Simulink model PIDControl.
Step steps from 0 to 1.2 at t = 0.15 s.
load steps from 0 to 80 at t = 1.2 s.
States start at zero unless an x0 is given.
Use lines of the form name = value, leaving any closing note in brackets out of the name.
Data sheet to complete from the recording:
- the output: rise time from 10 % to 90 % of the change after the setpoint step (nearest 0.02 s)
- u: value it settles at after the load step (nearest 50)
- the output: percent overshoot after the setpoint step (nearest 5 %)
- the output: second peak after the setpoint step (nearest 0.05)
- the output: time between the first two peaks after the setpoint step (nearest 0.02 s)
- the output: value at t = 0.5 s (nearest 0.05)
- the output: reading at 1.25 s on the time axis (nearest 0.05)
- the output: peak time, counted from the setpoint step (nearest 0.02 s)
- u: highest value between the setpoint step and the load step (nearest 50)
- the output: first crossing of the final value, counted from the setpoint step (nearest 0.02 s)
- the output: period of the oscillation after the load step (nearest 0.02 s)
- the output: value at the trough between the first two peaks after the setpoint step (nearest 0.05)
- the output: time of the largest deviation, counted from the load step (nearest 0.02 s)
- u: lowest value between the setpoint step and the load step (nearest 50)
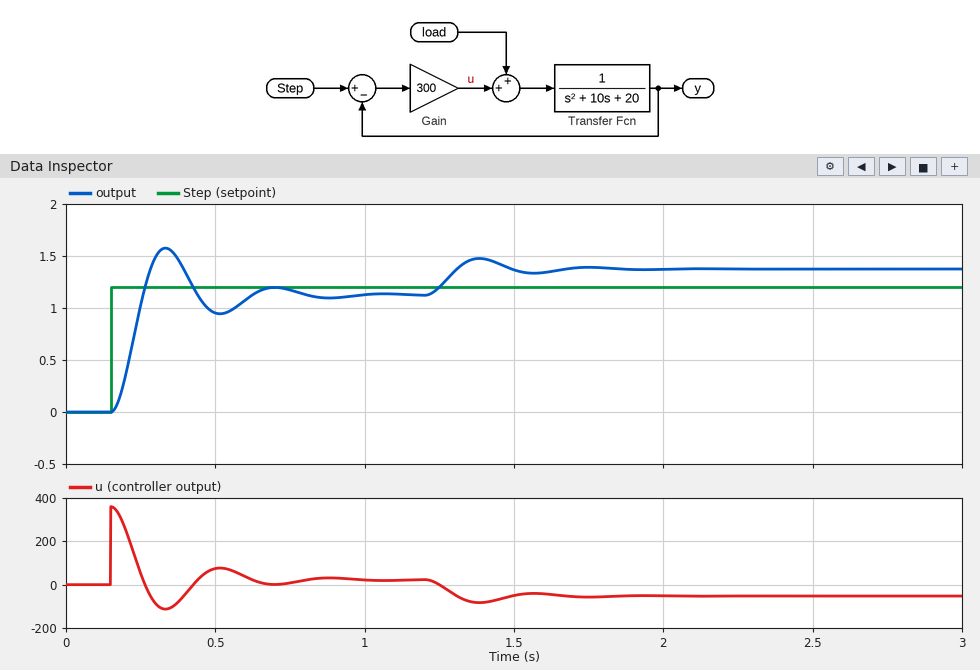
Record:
the output: rise time from 10 % to 90 % of the change after the setpoint step = 0.08 s
u: value it settles at after the load step = -50
the output: percent overshoot after the setpoint step = 40 %
the output: second peak after the setpoint step = 1.20
the output: time between the first two peaks after the setpoint step = 0.36 s
the output: value at t = 0.5 s = 0.95
the output: reading at 1.25 s on the time axis = 1.20
the output: peak time, counted from the setpoint step = 0.18 s
u: highest value between the setpoint step and the load step = 350
the output: first crossing of the final value, counted from the setpoint step = 0.10 s
the output: period of the oscillation after the load step = 0.36 s
the output: value at the trough between the first two peaks after the setpoint step = 0.95
the output: time of the largest deviation, counted from the load step = 0.18 s
u: lowest value between the setpoint step and the load step = -100
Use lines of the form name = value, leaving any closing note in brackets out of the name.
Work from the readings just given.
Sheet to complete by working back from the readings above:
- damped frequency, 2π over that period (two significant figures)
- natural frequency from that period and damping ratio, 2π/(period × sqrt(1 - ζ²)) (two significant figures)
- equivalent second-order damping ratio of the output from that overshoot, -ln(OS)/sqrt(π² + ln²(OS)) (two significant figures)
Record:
damped frequency, 2π over that period = 17 rad/s
natural frequency from that period and damping ratio, 2π/(period × sqrt(1 - ζ²)) = 18 rad/s
equivalent second-order damping ratio of the output from that overshoot, -ln(OS)/sqrt(π² + ln²(OS)) = 0.28
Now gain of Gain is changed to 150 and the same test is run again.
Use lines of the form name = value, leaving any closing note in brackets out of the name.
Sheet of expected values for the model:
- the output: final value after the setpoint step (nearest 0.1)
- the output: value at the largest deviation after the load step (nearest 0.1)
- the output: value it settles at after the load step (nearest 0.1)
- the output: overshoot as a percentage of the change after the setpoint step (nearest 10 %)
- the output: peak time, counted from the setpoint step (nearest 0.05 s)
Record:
the output: final value after the setpoint step = 1.1
the output: value at the largest deviation after the load step = 1.7
the output: value it settles at after the load step = 1.5
the output: overshoot as a percentage of the change after the setpoint step = 30 %
the output: peak time, counted from the setpoint step = 0.25 s
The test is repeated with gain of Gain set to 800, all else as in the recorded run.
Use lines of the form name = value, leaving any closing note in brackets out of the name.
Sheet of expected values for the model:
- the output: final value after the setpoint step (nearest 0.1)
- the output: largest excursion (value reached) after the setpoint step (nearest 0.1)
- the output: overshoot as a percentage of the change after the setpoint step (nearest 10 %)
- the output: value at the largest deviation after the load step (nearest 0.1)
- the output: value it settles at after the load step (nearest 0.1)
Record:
the output: final value after the setpoint step = 1.2
the output: largest excursion (value reached) after the setpoint step = 1.8
the output: overshoot as a percentage of the change after the setpoint step = 60 %
the output: value at the largest deviation after the load step = 1.3
the output: value it settles at after the load step = 1.3
